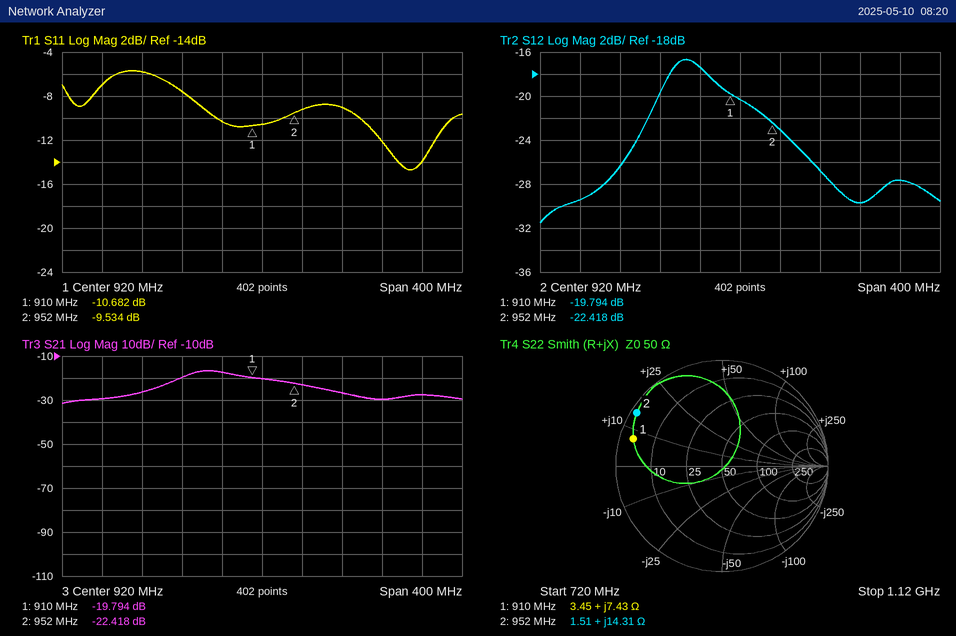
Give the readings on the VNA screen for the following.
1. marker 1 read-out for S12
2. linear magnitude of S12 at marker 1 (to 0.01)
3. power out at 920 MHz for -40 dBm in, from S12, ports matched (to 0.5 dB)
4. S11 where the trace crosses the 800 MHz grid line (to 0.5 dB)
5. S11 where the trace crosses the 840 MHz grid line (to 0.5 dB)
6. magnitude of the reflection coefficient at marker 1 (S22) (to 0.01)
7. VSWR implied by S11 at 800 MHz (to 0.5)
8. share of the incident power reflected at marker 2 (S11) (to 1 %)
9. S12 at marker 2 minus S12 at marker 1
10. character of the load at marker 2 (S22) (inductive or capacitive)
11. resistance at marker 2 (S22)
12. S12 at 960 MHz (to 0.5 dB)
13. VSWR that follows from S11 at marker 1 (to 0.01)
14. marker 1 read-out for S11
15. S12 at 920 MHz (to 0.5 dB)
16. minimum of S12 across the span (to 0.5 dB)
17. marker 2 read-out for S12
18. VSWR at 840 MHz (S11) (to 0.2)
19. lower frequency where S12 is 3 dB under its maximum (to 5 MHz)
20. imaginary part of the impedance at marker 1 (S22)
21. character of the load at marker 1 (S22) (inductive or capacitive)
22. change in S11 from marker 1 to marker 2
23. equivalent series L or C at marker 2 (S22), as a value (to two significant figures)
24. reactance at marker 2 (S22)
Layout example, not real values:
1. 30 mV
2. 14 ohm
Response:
1. -19.794 dB
2. 0.10
3. -60.5 dBm
4. -6.0 dB
5. -7.5 dB
6. 0.87
7. 3.0
8. 11 %
9. -2.624 dB
10. inductive
11. 1.51 Ω
12. -23.0 dB
13. 1.83
14. -10.682 dB
15. -20.5 dB
16. -31.5 dB
17. -22.418 dB
18. 2.4
19. 840 MHz
20. +7.43 Ω
21. inductive
22. 1.148 dB
23. 2.4 nH
24. +14.31 Ω
